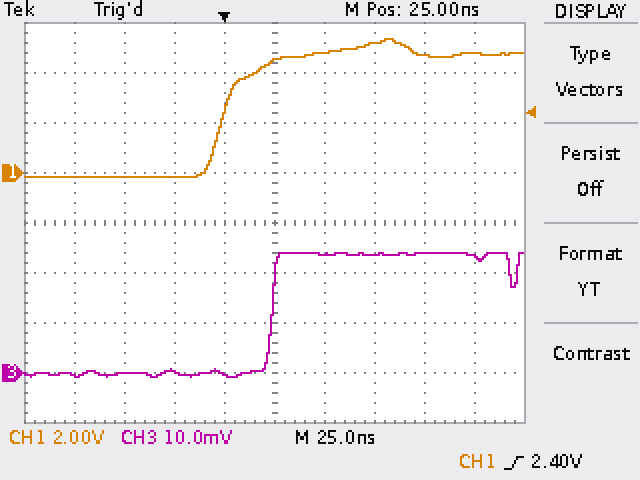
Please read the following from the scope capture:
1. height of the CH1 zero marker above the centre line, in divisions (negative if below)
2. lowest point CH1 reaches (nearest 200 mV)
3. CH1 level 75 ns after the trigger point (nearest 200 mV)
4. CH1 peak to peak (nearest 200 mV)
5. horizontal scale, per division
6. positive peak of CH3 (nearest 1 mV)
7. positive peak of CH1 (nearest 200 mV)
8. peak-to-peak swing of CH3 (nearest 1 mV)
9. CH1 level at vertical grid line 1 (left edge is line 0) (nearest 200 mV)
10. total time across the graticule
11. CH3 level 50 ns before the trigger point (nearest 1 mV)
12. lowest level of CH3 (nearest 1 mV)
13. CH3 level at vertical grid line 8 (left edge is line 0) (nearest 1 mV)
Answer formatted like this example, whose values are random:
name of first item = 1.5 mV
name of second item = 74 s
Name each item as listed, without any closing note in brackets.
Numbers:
height of the CH1 zero marker above the centre line, in divisions = +1.0 div
lowest point CH1 reaches = -200 mV
CH1 level 75 ns after the trigger point = 5.2 V
CH1 peak to peak = 5.6 V
horizontal scale, per division = 25 ns
positive peak of CH3 = 24 mV
positive peak of CH1 = 5.4 V
peak-to-peak swing of CH3 = 25 mV
CH1 level at vertical grid line 1 (left edge is line 0) = -200 mV
total time across the graticule = 250 ns
CH3 level 50 ns before the trigger point = 0 mV
lowest level of CH3 = -1 mV
CH3 level at vertical grid line 8 (left edge is line 0) = 24 mV
